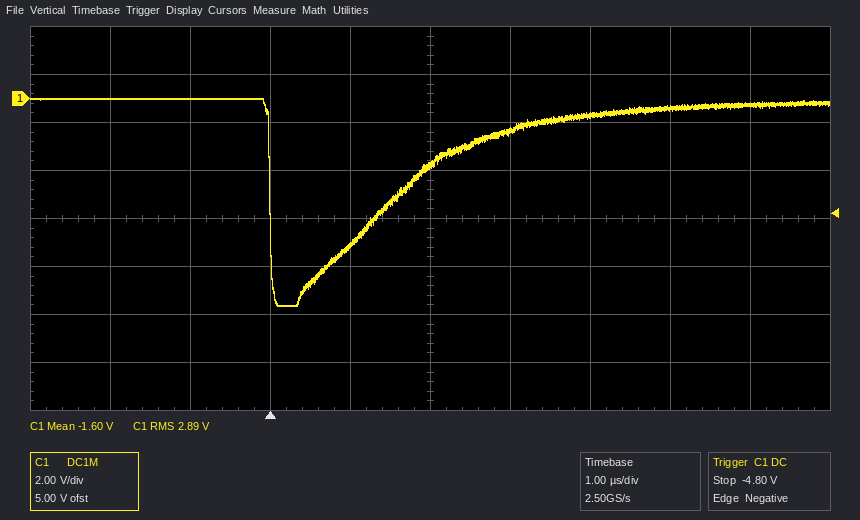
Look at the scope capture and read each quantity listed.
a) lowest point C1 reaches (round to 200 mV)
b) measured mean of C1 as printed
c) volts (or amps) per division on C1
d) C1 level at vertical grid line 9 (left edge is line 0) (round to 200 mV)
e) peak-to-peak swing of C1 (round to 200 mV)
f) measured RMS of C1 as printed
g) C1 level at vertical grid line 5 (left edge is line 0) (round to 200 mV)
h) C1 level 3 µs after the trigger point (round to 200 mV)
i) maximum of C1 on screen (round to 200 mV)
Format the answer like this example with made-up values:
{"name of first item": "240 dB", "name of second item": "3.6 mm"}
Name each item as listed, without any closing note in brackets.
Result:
{"lowest point C1 reaches": "-8.6 V", "measured mean of C1 as printed": "-1.60 V", "volts (or amps) per division on C1": "2 V", "C1 level at vertical grid line 9 (left edge is line 0)": "-200 mV", "peak-to-peak swing of C1": "8.6 V", "measured RMS of C1 as printed": "2.89 V", "C1 level at vertical grid line 5 (left edge is line 0)": "-2.8 V", "C1 level 3 µs after the trigger point": "-1.4 V", "maximum of C1 on screen": "0.0 V"}
